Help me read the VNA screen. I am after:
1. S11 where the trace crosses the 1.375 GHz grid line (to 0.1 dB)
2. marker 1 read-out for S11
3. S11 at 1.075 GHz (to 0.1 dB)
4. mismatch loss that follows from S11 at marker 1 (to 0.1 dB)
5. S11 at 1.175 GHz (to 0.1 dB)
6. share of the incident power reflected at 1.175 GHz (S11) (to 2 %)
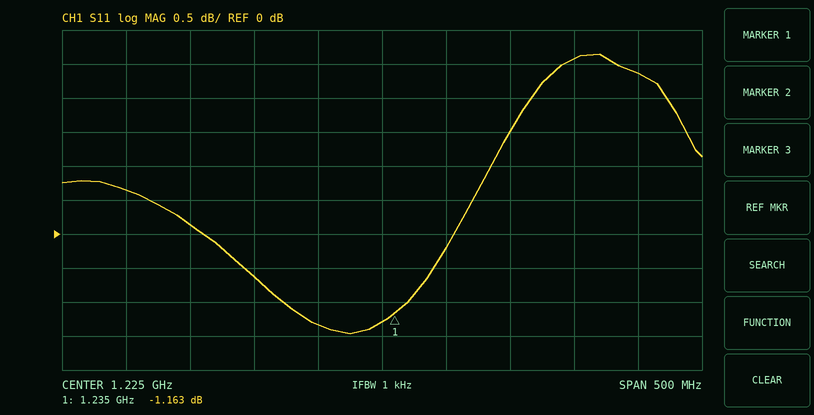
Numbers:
2.6 dB
-1.163 dB
0.1 dB
6.3 dB
-1.3 dB
74 %
